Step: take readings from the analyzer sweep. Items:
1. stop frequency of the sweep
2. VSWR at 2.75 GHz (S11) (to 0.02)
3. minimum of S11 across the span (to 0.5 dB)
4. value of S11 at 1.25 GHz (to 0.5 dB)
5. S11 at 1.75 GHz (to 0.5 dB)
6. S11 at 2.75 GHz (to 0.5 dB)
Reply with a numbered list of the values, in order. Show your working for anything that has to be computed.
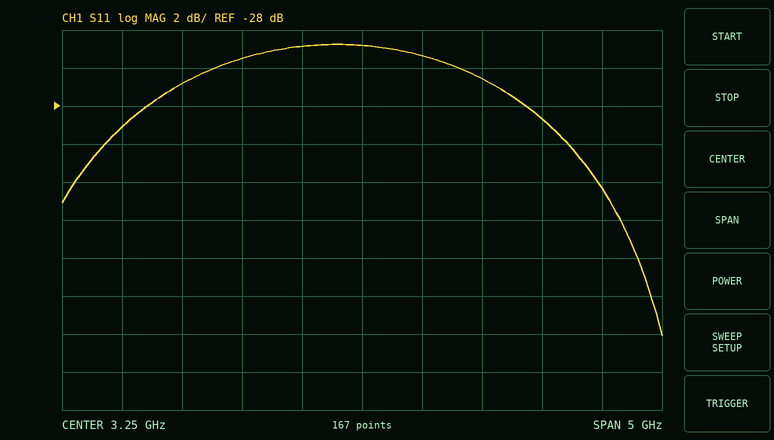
1. 5.75 GHz
2. |Γ| = 10^(-25/20) = 0.0562; VSWR = (1 + 0.0562)/(1 − 0.0562) ≈ 1.12
3. -40.0 dB
4. -29.0 dB
5. -27.0 dB
6. -25.0 dB
